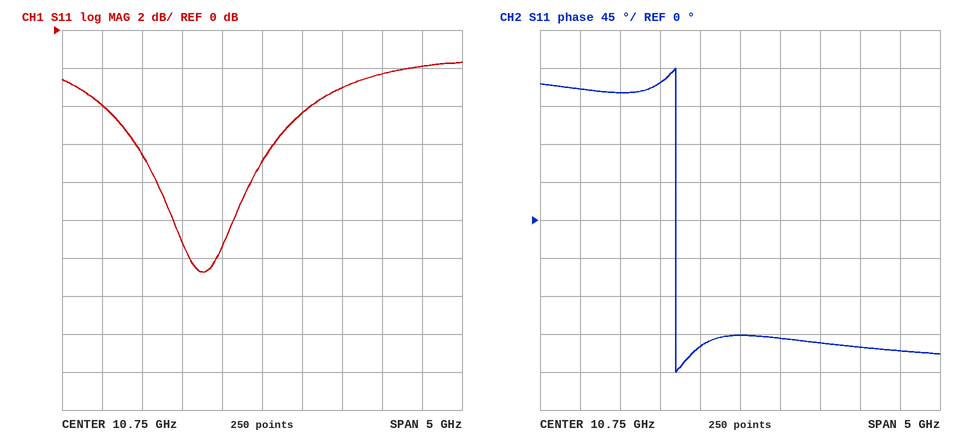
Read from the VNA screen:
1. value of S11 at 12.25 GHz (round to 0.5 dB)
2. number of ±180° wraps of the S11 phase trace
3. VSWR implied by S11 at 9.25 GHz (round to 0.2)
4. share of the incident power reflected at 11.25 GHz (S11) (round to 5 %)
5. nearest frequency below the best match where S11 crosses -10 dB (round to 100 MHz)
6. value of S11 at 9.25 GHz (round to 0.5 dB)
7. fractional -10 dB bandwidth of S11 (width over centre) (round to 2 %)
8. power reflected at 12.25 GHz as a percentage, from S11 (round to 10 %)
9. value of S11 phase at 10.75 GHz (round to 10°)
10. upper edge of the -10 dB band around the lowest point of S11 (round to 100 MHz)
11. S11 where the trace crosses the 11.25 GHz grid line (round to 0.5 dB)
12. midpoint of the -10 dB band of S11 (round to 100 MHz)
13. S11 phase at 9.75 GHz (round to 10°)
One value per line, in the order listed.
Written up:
-2.5 dB
1
2.8
35 %
9.6 GHz
-6.5 dB
8 %
60 %
-140°
10.4 GHz
-4.5 dB
10.0 GHz
160°
